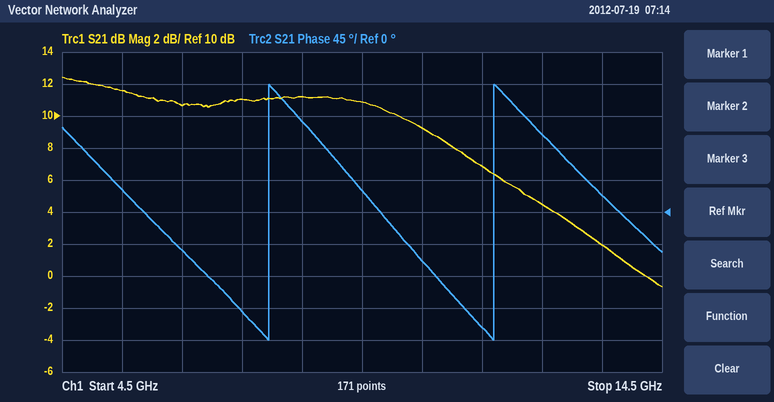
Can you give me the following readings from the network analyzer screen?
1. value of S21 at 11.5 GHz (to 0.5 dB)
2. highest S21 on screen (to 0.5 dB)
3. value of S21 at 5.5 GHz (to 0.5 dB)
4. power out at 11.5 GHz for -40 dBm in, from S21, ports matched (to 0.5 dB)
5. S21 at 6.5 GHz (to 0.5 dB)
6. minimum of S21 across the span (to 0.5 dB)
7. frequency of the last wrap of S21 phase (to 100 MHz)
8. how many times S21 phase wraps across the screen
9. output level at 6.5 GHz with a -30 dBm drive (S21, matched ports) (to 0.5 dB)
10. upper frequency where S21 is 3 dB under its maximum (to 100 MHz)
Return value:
7.0 dB
12.5 dB
11.5 dB
-33.0 dBm
10.5 dB
-0.5 dB
11.7 GHz
2
-19.5 dBm
10.4 GHz
